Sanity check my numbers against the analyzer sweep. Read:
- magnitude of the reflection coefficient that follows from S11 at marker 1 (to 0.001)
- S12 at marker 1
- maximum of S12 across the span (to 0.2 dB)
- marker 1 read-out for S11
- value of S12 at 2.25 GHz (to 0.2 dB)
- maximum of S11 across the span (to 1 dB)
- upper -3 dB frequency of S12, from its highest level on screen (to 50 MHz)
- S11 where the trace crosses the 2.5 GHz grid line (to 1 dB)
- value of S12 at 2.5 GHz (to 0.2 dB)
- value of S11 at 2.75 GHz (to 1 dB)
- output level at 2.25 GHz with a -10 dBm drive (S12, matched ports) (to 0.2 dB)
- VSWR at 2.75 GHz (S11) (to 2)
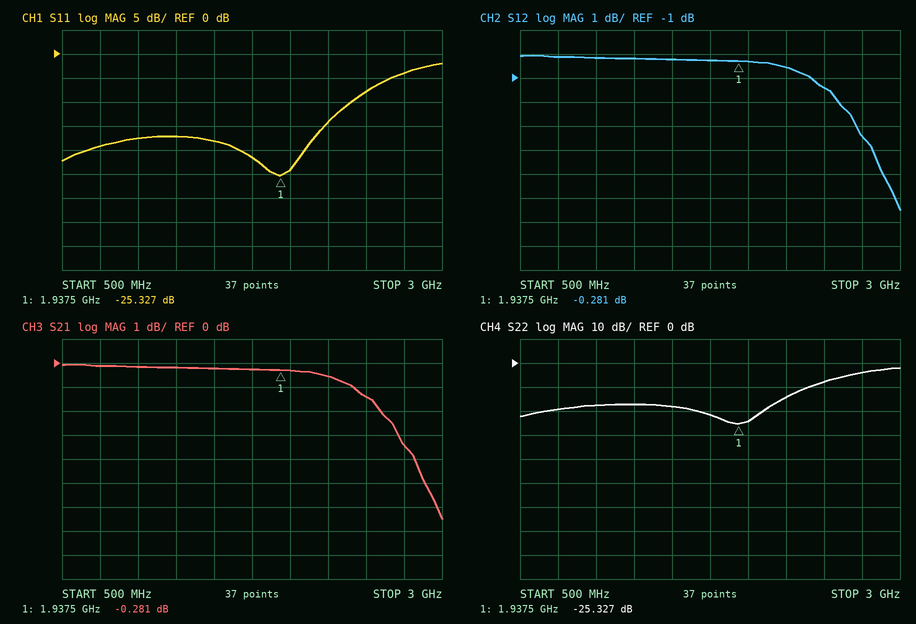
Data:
0.054
-0.281 dB
0.0 dB
-25.327 dB
-0.6 dB
-2 dB
2.70 GHz
-8 dB
-1.4 dB
-4 dB
-10.6 dBm
4
